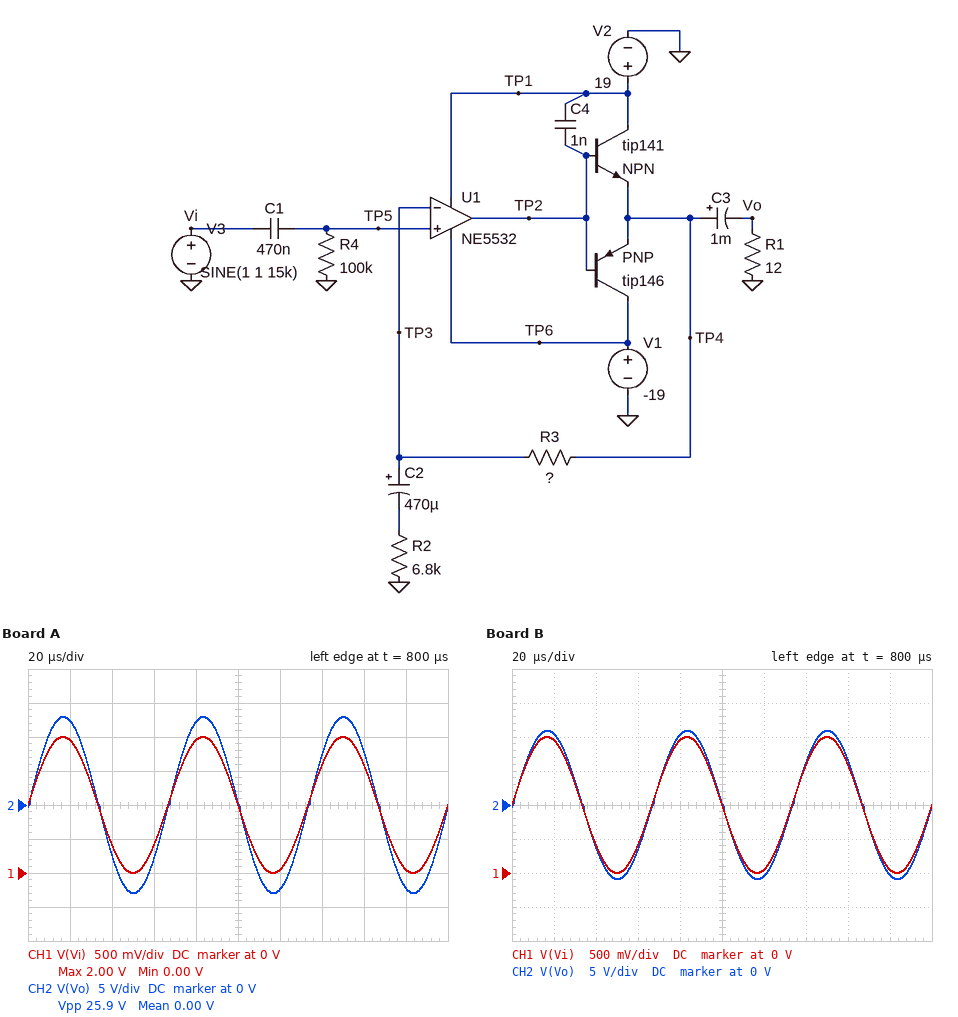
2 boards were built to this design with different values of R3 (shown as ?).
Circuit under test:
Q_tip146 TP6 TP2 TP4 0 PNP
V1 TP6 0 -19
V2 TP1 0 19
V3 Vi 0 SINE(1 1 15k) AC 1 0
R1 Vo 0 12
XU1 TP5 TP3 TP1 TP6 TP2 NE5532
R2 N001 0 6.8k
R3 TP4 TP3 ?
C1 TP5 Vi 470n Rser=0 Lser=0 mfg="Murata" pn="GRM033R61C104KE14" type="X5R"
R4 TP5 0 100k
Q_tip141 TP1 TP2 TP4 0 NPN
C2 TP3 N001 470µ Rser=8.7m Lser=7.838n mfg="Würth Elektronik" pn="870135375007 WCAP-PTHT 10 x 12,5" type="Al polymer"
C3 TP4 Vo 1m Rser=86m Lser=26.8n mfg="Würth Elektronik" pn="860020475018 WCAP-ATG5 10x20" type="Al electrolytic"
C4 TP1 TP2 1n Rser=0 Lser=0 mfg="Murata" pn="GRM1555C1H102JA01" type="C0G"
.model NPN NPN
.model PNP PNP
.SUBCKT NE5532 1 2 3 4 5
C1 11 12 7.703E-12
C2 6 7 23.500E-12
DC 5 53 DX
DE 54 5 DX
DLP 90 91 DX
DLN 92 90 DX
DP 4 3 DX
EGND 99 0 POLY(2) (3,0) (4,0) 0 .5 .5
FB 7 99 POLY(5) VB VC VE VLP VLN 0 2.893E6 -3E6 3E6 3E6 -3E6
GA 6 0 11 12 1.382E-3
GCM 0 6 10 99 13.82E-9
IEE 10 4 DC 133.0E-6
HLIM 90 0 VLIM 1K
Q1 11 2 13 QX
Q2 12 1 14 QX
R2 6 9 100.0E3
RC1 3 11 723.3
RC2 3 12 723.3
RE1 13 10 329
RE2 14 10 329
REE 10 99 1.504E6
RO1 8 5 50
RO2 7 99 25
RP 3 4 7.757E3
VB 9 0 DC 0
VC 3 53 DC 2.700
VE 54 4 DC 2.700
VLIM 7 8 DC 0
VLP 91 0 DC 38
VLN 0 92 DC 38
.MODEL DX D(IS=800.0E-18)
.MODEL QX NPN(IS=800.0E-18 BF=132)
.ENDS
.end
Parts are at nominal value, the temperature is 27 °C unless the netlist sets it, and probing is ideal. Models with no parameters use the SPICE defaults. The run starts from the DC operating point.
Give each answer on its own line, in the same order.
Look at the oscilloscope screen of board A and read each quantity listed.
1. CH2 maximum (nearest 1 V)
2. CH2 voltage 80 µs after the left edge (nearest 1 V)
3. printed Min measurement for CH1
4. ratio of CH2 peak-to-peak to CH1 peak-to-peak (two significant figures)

13 V
12 V
0.00 V
13
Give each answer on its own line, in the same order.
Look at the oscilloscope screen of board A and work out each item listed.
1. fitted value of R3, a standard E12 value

82 kΩ
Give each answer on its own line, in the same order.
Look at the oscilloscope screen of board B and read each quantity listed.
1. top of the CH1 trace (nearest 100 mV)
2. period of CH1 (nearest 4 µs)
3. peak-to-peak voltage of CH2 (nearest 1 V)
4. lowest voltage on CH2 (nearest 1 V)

2.0 V
68 µs
22 V
-11 V
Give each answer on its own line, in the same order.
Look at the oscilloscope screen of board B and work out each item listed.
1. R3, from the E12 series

68 kΩ
